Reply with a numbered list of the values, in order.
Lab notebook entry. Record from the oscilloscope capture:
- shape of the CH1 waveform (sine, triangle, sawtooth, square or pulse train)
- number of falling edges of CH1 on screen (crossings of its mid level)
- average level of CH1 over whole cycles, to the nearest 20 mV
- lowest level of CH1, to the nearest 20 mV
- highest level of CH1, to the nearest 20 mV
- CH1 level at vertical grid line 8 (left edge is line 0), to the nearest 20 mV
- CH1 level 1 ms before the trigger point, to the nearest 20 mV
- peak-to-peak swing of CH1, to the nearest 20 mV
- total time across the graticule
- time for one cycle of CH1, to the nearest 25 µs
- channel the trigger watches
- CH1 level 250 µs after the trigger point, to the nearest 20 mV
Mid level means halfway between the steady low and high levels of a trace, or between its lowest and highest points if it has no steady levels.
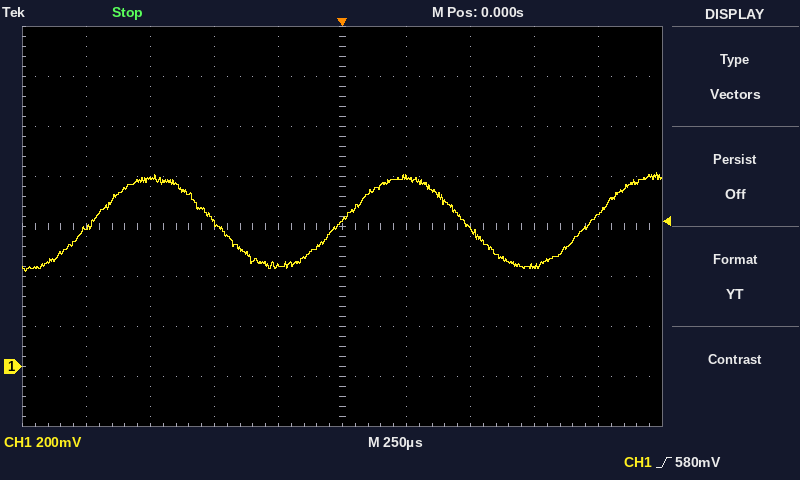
1. sine
2. 2
3. 580 mV
4. 380 mV
5. 780 mV
6. 400 mV
7. 560 mV
8. 400 mV
9. 2.5 ms
10. 975 µs
11. CH1
12. 760 mV
